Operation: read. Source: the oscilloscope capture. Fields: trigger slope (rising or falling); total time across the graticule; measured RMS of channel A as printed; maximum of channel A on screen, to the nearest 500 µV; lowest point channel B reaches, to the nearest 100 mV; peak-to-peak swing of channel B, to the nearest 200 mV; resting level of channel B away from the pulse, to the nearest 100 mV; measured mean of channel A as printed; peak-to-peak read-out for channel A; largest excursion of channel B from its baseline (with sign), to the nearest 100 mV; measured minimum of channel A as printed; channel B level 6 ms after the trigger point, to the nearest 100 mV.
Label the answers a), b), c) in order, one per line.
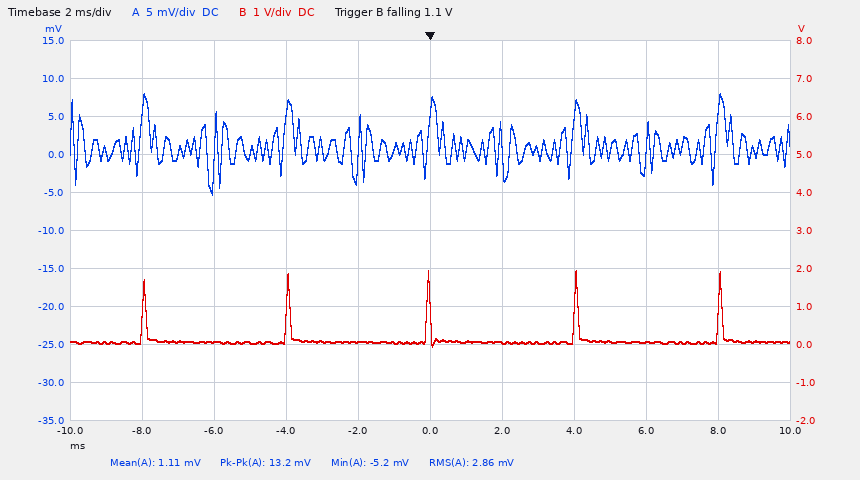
a) falling
b) 20 ms
c) 2.86 mV
d) 8.0 mV
e) -100 mV
f) 2.0 V
g) 100 mV
h) 1.11 mV
i) 13.2 mV
j) +1.9 V
k) -5.2 mV
l) 100 mV
